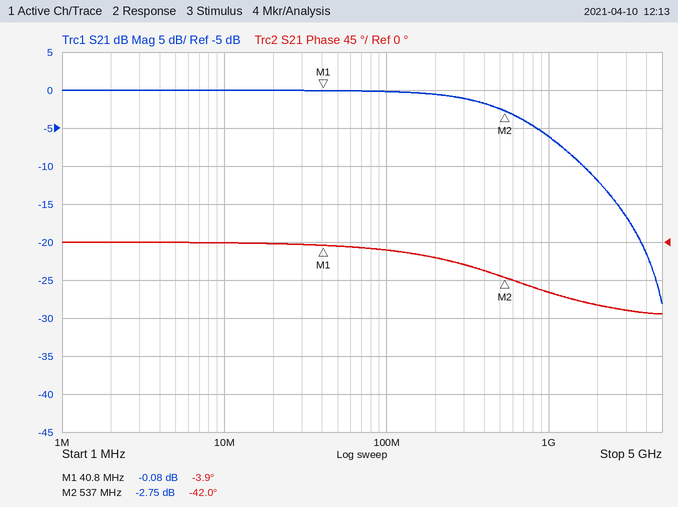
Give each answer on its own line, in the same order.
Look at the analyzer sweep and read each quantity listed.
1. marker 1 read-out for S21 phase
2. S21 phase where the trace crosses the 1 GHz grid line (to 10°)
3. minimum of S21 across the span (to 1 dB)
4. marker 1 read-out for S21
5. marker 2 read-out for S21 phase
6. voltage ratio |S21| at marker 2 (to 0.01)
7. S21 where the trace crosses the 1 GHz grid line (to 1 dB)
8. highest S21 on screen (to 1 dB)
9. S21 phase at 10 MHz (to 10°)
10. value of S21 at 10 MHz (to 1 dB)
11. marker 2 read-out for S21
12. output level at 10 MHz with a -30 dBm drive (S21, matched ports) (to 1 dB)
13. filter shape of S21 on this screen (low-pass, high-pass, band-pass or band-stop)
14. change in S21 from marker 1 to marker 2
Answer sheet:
-3.9°
-60°
-28 dB
-0.08 dB
-42.0°
0.73
-6 dB
0 dB
0°
0 dB
-2.75 dB
-30 dBm
low-pass
-2.67 dB
